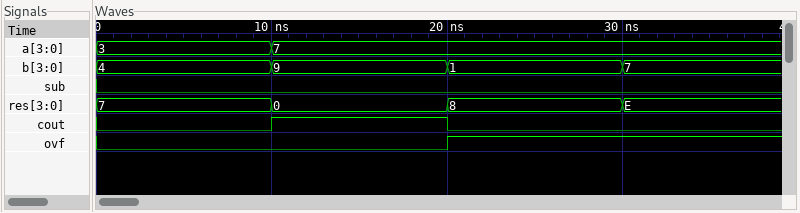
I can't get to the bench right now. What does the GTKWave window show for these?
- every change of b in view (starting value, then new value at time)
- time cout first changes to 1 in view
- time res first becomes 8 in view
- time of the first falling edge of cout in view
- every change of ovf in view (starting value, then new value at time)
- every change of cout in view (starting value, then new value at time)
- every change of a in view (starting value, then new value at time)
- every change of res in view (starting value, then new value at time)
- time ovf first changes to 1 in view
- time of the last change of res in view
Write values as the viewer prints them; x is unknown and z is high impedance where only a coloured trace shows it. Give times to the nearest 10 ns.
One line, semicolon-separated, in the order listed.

4, 9 at 10 ns, 1 at 20 ns, 7 at 30 ns; 10 ns; 20 ns; 20 ns; 0, 1 at 20 ns; 0, 1 at 10 ns, 0 at 20 ns; 3, 7 at 10 ns; 7, 0 at 10 ns, 8 at 20 ns, E at 30 ns; 20 ns; 30 ns
